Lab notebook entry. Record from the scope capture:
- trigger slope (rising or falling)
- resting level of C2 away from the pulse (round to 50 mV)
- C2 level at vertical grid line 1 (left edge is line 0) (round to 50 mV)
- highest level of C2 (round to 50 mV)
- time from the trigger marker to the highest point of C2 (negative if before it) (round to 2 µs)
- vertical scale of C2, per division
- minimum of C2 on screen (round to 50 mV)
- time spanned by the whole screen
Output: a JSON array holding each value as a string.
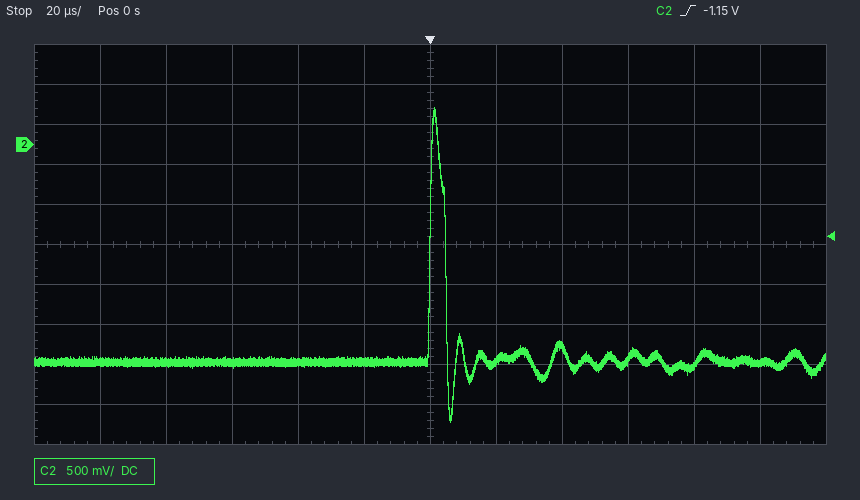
["rising", "-2.70 V", "-2.70 V", "450 mV", "+2 µs", "500 mV", "-3.45 V", "240 µs"]
